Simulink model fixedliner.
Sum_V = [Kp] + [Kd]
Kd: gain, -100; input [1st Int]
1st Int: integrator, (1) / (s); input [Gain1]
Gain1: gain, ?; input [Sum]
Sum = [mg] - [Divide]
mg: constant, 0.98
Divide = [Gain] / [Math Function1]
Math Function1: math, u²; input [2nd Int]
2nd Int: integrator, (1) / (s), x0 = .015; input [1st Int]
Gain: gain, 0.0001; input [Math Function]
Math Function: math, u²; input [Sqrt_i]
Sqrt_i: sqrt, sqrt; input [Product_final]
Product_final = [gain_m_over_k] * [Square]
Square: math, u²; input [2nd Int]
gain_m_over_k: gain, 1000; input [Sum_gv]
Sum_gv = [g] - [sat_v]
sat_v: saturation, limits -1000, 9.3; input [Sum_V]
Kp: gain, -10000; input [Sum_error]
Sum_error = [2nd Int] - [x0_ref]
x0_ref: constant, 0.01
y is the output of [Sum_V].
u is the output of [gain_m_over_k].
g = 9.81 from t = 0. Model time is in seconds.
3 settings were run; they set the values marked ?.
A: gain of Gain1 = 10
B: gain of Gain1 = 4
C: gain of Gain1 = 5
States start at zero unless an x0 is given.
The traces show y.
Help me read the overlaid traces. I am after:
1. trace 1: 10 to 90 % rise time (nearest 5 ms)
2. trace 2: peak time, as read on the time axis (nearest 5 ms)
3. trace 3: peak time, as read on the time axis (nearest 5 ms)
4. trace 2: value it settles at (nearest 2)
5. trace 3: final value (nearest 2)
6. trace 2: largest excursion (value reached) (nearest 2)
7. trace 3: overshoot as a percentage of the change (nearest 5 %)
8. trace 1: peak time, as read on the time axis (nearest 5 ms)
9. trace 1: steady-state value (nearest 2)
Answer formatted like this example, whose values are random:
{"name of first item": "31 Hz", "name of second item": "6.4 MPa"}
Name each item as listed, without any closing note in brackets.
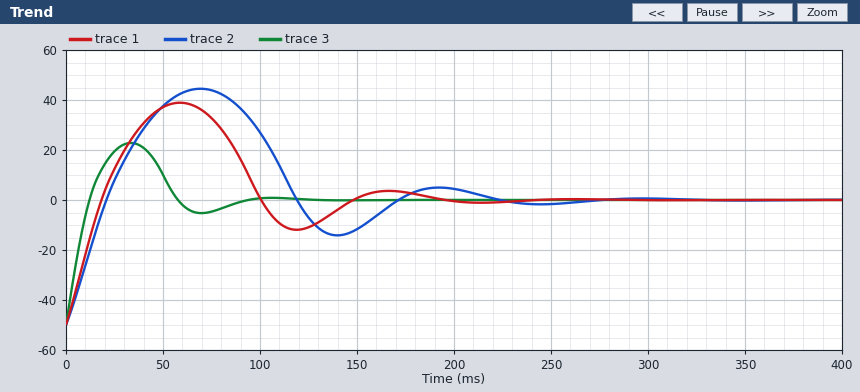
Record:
{"trace 1: 10 to 90 % rise time": "15 ms", "trace 2: peak time, as read on the time axis": "70 ms", "trace 3: peak time, as read on the time axis": "35 ms", "trace 2: value it settles at": "0", "trace 3: final value": "0", "trace 2: largest excursion (value reached)": "44", "trace 3: overshoot as a percentage of the change": "45 %", "trace 1: peak time, as read on the time axis": "60 ms", "trace 1: steady-state value": "0"}
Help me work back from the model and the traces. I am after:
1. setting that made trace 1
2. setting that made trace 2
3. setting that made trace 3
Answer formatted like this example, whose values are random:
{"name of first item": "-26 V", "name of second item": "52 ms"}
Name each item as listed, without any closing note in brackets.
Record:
{"setting that made trace 1": "C", "setting that made trace 2": "B", "setting that made trace 3": "A"}
